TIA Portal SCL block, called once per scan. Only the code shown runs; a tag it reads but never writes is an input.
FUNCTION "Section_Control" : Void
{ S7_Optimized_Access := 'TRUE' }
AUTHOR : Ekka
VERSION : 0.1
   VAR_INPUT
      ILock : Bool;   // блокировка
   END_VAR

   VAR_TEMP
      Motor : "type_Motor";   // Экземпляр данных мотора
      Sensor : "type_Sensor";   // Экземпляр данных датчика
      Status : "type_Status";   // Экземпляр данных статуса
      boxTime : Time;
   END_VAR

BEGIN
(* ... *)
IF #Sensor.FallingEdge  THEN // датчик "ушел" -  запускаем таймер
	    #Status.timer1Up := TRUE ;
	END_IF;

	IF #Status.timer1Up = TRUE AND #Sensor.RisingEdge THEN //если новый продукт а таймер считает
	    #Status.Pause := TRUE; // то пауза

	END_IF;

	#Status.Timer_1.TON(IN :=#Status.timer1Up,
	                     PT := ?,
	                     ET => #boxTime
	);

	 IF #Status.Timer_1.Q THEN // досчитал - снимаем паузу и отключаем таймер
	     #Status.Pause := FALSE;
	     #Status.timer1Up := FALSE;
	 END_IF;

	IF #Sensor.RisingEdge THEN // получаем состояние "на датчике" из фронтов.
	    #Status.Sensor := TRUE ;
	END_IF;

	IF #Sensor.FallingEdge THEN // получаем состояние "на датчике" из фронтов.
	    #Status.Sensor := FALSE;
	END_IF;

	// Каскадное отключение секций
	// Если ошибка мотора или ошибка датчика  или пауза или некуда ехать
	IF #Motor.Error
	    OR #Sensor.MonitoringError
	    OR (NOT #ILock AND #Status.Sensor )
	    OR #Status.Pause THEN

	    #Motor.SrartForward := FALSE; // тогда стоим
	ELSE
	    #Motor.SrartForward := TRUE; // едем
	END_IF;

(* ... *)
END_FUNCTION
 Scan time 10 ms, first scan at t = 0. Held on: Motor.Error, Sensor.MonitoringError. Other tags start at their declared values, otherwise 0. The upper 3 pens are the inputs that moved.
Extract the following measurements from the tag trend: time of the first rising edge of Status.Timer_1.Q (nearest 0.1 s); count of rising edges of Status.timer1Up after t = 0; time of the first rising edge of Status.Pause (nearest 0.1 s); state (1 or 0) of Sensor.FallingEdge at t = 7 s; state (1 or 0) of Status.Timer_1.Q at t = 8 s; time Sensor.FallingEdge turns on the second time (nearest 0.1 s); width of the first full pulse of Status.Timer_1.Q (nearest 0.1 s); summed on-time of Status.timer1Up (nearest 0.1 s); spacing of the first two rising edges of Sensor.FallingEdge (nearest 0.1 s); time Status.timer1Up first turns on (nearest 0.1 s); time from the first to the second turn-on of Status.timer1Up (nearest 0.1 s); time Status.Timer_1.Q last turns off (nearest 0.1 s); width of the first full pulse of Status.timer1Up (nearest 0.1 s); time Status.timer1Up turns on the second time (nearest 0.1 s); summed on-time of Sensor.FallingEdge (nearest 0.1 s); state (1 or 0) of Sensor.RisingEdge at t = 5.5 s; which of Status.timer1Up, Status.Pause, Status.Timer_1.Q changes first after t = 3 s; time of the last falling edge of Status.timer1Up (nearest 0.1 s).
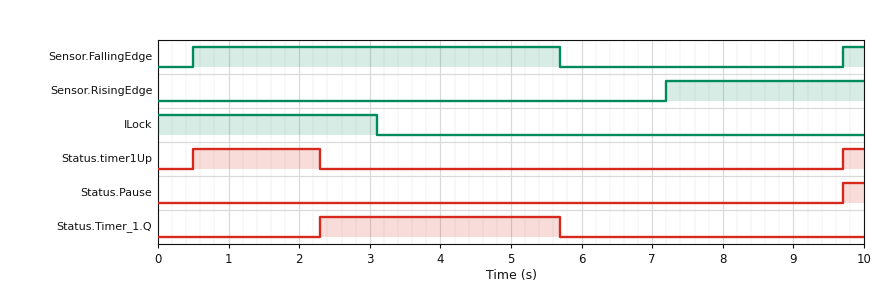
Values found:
2.3 s
2
9.7 s
0
0
9.7 s
3.4 s
2.1 s
9.2 s
0.5 s
9.2 s
5.7 s
1.8 s
9.7 s
5.5 s
0
Status.Timer_1.Q
2.3 s
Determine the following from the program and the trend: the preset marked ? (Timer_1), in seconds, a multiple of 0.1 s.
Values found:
1.8 s
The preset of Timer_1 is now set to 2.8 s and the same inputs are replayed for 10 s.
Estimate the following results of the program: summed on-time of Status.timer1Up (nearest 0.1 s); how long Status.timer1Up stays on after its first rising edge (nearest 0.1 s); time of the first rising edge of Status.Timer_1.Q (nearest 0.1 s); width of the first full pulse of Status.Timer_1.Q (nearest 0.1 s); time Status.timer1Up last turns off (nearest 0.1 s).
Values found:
3.1 s
2.8 s
3.3 s
2.4 s
3.3 s
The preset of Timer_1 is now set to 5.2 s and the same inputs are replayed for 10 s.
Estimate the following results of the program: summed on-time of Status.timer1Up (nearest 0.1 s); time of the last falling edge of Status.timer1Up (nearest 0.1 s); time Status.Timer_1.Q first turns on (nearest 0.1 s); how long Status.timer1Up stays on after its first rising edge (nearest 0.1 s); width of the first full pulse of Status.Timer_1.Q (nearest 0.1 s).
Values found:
5.5 s
5.7 s
5.7 s
5.2 s
0.0 s
